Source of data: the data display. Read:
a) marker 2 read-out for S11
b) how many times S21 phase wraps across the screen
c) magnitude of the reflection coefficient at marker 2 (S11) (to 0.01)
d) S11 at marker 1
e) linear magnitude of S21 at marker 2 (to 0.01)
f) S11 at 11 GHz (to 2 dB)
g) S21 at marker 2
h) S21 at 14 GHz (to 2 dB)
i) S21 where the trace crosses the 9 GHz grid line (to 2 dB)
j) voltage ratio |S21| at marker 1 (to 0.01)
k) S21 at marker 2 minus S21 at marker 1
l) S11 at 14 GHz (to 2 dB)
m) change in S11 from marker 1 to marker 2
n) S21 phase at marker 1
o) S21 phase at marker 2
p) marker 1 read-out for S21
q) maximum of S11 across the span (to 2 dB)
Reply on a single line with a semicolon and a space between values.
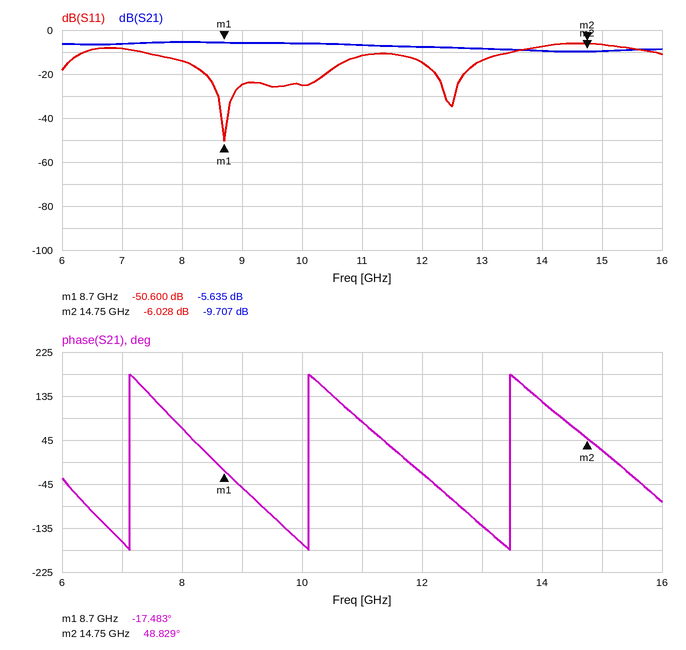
-6.028 dB; 3; 0.50; -50.600 dB; 0.33; -12 dB; -9.707 dB; -10 dB; -6 dB; 0.52; -4.072 dB; -8 dB; 44.572 dB; -17.483°; 48.829°; -5.635 dB; -6 dB
